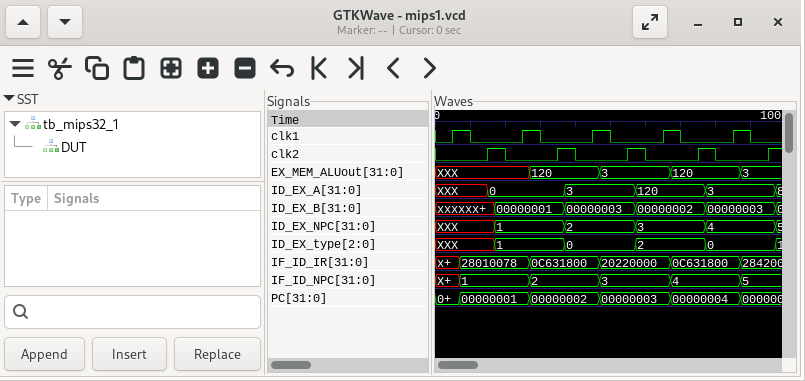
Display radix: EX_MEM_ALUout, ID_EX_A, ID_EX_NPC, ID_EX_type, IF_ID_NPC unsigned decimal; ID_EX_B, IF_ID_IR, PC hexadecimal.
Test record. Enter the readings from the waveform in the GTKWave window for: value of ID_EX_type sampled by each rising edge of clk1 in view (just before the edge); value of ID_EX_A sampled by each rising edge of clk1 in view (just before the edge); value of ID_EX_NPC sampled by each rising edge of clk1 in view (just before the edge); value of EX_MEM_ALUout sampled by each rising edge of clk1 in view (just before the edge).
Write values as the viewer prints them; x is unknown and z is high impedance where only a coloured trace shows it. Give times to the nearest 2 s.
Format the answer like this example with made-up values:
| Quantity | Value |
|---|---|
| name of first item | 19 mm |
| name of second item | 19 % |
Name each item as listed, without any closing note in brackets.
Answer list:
| Quantity | Value |
|---|---|
| value of ID_EX_type sampled by each rising edge of clk1 in view | XXX, 1, 0, 2, 0 |
| value of ID_EX_A sampled by each rising edge of clk1 in view | XXX, 0, 3, 120, 3 |
| value of ID_EX_NPC sampled by each rising edge of clk1 in view | XXX, 1, 2, 3, 4 |
| value of EX_MEM_ALUout sampled by each rising edge of clk1 in view | XXX, XXX, 120, 3, 120 |
